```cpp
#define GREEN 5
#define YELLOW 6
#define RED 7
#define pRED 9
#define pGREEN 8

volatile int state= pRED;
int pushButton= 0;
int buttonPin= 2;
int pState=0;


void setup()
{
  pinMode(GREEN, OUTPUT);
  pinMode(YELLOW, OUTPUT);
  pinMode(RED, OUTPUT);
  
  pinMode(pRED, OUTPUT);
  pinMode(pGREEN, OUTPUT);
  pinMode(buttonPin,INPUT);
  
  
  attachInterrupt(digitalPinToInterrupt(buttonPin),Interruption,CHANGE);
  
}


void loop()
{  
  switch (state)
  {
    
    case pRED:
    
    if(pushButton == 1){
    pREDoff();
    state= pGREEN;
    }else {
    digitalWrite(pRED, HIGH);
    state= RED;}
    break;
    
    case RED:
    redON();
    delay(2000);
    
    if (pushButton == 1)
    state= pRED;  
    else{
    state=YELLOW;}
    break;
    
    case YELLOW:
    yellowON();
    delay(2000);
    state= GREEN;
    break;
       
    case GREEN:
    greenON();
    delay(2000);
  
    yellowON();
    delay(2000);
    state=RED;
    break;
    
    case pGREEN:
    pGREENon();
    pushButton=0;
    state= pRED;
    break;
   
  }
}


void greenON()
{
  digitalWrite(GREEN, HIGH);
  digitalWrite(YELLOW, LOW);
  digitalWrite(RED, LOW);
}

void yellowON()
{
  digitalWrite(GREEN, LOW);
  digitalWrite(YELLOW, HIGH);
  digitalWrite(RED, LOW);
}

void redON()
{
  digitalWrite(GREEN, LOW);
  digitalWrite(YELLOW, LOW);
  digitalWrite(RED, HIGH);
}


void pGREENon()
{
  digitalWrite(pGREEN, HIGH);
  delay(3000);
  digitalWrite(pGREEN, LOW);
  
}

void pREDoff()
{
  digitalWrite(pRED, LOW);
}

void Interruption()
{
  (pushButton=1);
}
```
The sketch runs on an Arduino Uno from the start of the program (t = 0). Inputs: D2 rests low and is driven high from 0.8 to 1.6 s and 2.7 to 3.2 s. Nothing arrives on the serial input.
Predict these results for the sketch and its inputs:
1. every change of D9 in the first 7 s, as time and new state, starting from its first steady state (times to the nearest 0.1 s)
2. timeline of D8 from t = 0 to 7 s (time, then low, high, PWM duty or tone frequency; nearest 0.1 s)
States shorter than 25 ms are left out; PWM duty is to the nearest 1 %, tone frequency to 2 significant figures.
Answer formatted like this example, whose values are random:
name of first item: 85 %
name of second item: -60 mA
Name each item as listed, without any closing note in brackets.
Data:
every change of D9 in the first 7 s, as time and new state, starting from its first steady state: 0 s high; 2 s low; 5 s high
timeline of D8 from t = 0 to 7 s: 0 s low; 2 s high; 5 s low
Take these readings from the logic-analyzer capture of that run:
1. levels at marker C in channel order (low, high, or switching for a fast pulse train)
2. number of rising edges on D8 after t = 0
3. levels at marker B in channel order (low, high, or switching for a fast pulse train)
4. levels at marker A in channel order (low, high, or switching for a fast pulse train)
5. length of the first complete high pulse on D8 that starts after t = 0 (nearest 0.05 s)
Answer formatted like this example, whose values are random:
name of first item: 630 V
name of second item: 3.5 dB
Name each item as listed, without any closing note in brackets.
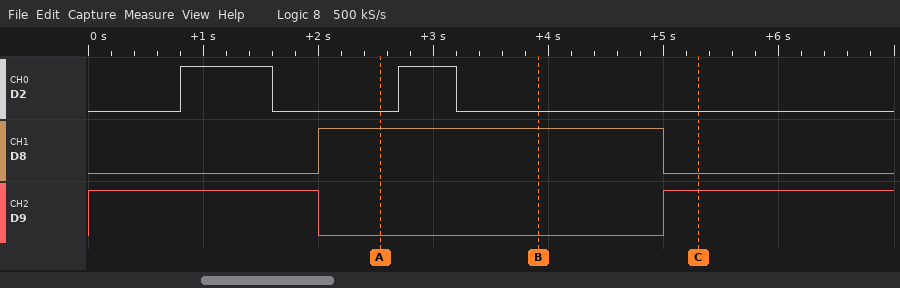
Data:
levels at marker C in channel order: D2 low, D8 low, D9 high
number of rising edges on D8 after t = 0: 1
levels at marker B in channel order: D2 low, D8 high, D9 low
levels at marker A in channel order: D2 low, D8 high, D9 low
length of the first complete high pulse on D8 that starts after t = 0: 3.00 s
